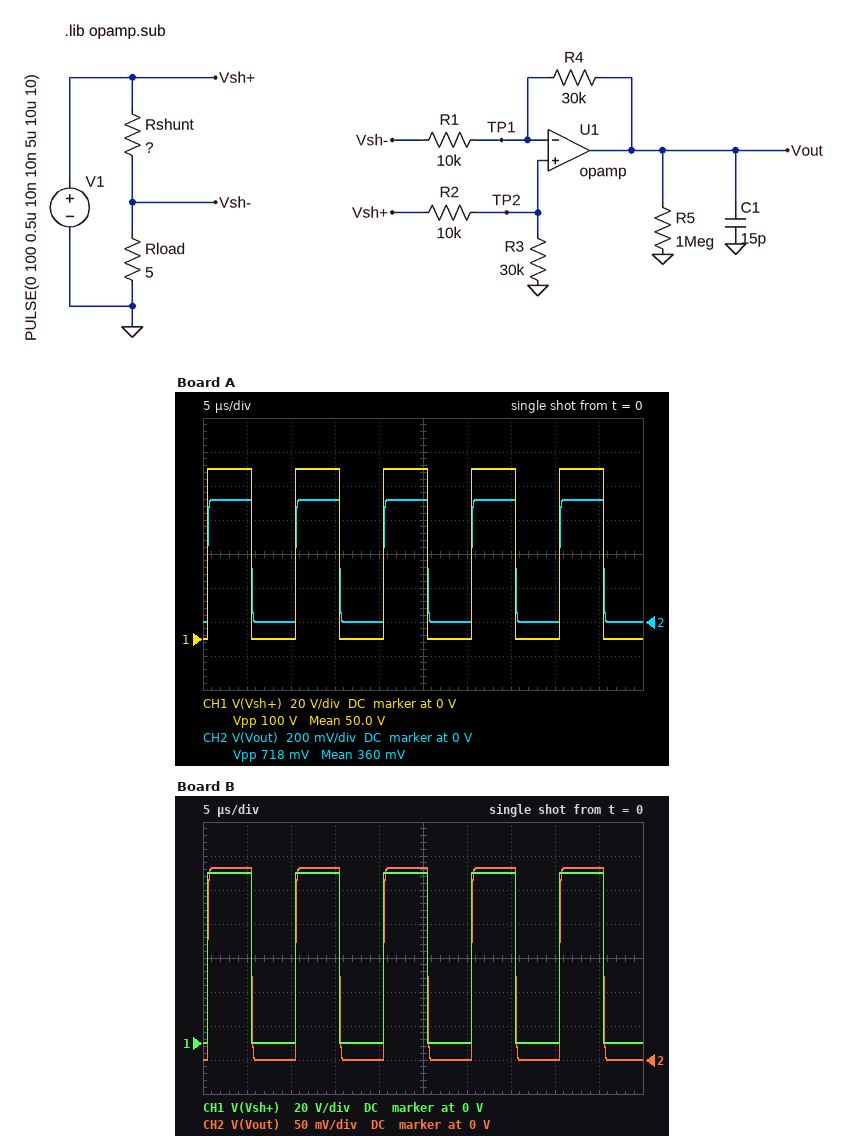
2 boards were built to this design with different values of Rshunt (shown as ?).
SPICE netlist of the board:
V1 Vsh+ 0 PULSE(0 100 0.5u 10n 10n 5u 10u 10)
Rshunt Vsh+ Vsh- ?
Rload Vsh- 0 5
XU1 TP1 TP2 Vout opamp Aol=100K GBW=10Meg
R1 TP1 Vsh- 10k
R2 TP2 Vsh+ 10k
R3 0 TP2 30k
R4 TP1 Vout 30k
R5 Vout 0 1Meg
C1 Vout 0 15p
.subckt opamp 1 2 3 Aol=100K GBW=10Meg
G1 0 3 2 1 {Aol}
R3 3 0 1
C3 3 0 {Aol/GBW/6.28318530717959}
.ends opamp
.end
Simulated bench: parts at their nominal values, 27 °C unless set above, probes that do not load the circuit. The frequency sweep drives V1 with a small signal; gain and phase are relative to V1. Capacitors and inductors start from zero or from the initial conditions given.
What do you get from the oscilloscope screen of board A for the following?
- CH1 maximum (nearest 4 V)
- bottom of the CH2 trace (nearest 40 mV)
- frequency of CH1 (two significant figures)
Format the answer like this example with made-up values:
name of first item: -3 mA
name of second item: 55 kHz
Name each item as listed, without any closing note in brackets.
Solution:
CH1 maximum: 100 V
bottom of the CH2 trace: 0 V
frequency of CH1: 100 kHz
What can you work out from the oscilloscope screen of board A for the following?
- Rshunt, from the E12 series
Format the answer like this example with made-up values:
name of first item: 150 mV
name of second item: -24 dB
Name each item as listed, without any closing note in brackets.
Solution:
Rshunt, from the E12 series: 0.012 Ω
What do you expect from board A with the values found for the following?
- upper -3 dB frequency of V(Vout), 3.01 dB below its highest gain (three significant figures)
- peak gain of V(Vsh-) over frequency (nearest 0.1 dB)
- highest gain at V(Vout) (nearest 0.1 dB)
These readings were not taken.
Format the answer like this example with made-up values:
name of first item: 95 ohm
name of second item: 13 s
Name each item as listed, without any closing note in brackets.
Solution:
upper -3 dB frequency of V(Vout), 3.01 dB below its highest gain: 2.50 MHz
peak gain of V(Vsh-) over frequency: 0 dB
highest gain at V(Vout): -42.9 dB
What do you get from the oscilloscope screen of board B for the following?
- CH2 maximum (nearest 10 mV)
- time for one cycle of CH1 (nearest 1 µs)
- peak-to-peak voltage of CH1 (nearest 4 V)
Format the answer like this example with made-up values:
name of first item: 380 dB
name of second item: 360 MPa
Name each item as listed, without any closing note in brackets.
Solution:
CH2 maximum: 280 mV
time for one cycle of CH1: 10 µs
peak-to-peak voltage of CH1: 100 V
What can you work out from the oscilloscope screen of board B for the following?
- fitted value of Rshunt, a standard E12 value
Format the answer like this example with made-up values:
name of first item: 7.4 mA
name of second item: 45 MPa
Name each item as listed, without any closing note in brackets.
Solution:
fitted value of Rshunt, a standard E12 value: 4.7 mΩ
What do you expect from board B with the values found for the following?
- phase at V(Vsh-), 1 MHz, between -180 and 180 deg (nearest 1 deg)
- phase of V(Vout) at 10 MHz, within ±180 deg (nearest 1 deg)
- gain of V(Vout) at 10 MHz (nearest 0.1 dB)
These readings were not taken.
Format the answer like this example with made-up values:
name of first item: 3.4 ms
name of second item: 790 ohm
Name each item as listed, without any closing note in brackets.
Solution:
phase at V(Vsh-), 1 MHz, between -180 and 180 deg: 0 deg
phase of V(Vout) at 10 MHz, within ±180 deg: -76 deg
gain of V(Vout) at 10 MHz: -63.3 dB
